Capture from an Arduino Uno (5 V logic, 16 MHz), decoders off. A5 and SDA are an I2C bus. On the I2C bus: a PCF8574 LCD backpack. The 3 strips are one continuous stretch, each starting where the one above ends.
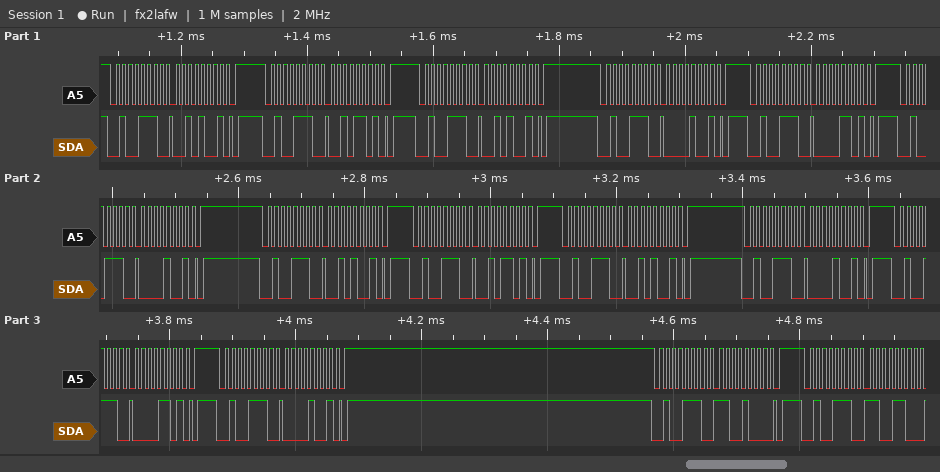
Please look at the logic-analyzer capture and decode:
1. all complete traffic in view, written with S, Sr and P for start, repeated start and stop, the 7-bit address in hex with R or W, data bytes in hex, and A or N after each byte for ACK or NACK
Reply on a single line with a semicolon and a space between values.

S 27W A 29 A P S 27W A 2D A P S 27W A 29 A P S 27W A 09 A P S 27W A 0D A P S 27W A 09 A P S 27W A 29 A P S 27W A 2D A P S 27W A 29 A P S 27W A 09 A P S 27W A 0D A P S 27W A 09 A P S 27W A C8 A P S 27W A CC A
